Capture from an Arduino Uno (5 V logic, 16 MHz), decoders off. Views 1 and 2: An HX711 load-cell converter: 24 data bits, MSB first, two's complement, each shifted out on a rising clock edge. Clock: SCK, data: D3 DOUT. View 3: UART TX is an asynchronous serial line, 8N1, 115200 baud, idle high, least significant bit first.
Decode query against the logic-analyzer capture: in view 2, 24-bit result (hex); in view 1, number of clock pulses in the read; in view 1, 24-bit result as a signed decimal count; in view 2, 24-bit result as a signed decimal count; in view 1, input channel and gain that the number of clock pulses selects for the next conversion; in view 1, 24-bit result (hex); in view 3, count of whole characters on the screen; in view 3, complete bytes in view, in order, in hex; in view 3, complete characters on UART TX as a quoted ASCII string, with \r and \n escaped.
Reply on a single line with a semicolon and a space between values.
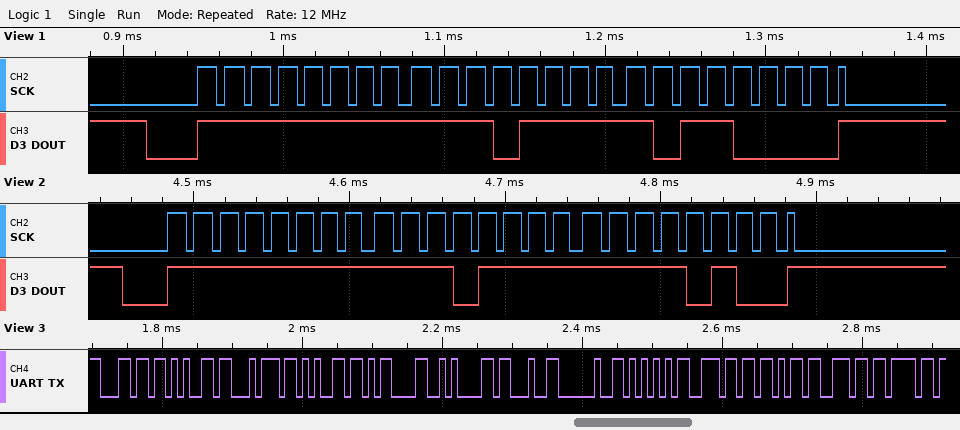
0xFFEFF4; 25; -4176; -4108; channel A, gain 128; 0xFFEFB0; 13; 6C 65 74 65 0D 0A 23 20 55 6E 6B 6E 6F; "lete\r\n# Unkno"
